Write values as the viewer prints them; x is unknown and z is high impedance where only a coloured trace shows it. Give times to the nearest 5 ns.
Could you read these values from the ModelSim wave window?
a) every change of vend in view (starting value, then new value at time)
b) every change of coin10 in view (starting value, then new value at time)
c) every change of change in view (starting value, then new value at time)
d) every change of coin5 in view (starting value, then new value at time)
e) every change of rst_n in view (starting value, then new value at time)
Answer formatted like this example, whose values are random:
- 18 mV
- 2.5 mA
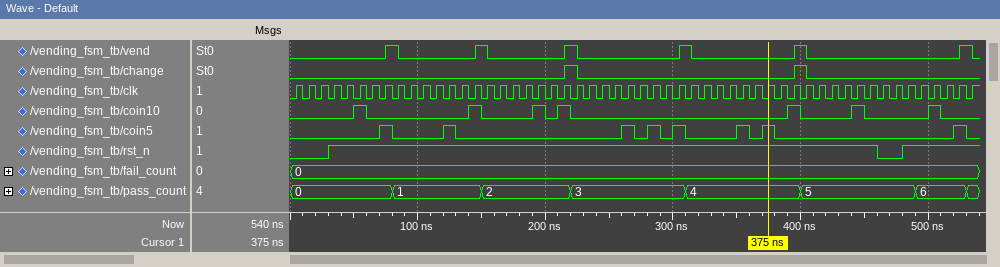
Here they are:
- 0, 1 at 75 ns, 0 at 85 ns, 1 at 145 ns, 0 at 155 ns, 1 at 215 ns, 0 at 225 ns, 1 at 305 ns, 0 at 315 ns, 1 at 395 ns, 0 at 405 ns, 1 at 525 ns, 0 at 535 ns
- 0, 1 at 50 ns, 0 at 60 ns, 1 at 140 ns, 0 at 150 ns, 1 at 190 ns, 0 at 200 ns, 1 at 210 ns, 0 at 220 ns, 1 at 390 ns, 0 at 400 ns, 1 at 440 ns, 0 at 450 ns, 1 at 500 ns, 0 at 510 ns
- 0, 1 at 215 ns, 0 at 225 ns, 1 at 395 ns, 0 at 405 ns
- 0, 1 at 70 ns, 0 at 80 ns, 1 at 120 ns, 0 at 130 ns, 1 at 260 ns, 0 at 270 ns, 1 at 280 ns, 0 at 290 ns, 1 at 300 ns, 0 at 310 ns, 1 at 350 ns, 0 at 360 ns, 1 at 370 ns, 0 at 380 ns, 1 at 520 ns, 0 at 530 ns
- 0, 1 at 30 ns, 0 at 460 ns, 1 at 480 ns
